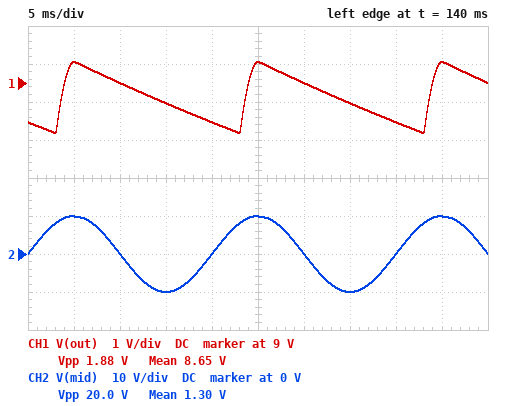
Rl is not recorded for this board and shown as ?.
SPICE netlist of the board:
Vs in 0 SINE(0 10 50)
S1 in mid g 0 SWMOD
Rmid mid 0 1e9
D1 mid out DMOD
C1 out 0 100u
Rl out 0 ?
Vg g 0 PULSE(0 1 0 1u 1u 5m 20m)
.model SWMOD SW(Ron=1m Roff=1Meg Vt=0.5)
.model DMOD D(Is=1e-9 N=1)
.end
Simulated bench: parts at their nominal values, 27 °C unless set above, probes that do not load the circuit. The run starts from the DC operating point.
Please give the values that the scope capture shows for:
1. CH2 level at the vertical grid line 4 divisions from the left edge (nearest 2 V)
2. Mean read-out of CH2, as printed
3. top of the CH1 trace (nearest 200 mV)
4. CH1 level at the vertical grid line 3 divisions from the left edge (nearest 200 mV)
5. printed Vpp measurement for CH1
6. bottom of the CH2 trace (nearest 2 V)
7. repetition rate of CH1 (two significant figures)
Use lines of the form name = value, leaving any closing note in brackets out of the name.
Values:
CH2 level at the vertical grid line 4 divisions from the left edge = 0 V
Mean read-out of CH2, as printed = 1.30 V
top of the CH1 trace = 9.6 V
CH1 level at the vertical grid line 3 divisions from the left edge = 8.4 V
printed Vpp measurement for CH1 = 1.88 V
bottom of the CH2 trace = -10 V
repetition rate of CH1 = 50 Hz
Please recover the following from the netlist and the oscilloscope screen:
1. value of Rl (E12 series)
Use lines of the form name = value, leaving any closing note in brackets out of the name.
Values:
value of Rl = 820 Ω
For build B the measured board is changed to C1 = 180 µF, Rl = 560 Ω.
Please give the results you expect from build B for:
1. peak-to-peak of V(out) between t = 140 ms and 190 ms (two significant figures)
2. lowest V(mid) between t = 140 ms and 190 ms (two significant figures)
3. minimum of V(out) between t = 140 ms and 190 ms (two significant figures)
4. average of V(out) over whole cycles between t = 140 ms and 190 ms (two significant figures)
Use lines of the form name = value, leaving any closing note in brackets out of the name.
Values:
peak-to-peak of V(out) between t = 140 ms and 190 ms = 1.6 V
lowest V(mid) between t = 140 ms and 190 ms = -10 V
minimum of V(out) between t = 140 ms and 190 ms = 8.0 V
average of V(out) over whole cycles between t = 140 ms and 190 ms = 8.8 V
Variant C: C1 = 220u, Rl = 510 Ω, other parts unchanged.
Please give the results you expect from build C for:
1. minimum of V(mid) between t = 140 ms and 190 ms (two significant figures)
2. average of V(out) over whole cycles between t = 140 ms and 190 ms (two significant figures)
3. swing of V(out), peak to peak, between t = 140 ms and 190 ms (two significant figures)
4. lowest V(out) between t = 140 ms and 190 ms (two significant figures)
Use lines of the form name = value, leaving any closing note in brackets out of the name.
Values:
minimum of V(mid) between t = 140 ms and 190 ms = -10 V
average of V(out) over whole cycles between t = 140 ms and 190 ms = 8.8 V
swing of V(out), peak to peak, between t = 140 ms and 190 ms = 1.4 V
lowest V(out) between t = 140 ms and 190 ms = 8.1 V
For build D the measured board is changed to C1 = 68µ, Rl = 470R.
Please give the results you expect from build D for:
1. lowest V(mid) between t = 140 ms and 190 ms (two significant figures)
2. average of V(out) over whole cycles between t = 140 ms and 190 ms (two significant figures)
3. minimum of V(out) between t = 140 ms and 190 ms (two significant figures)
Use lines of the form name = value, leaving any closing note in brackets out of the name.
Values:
lowest V(mid) between t = 140 ms and 190 ms = -10 V
average of V(out) over whole cycles between t = 140 ms and 190 ms = 7.5 V
minimum of V(out) between t = 140 ms and 190 ms = 5.6 V
